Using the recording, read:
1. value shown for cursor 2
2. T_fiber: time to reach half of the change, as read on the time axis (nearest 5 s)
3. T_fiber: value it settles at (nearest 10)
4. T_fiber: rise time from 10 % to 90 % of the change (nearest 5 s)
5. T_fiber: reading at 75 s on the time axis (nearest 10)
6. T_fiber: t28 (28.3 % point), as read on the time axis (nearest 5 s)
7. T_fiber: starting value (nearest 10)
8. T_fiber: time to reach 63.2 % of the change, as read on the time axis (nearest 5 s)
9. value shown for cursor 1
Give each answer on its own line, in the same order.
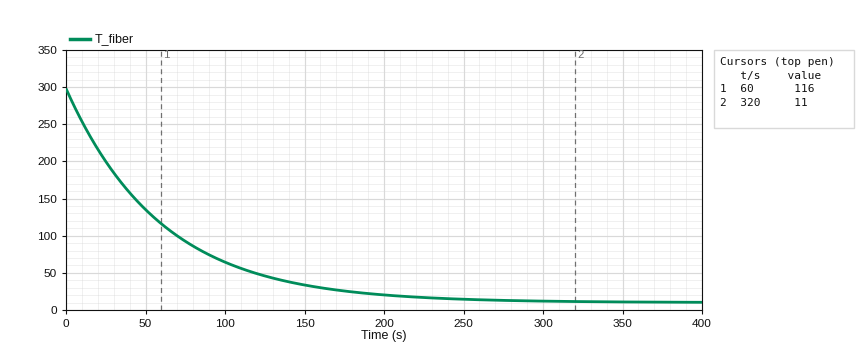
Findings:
11
40 s
10
130 s
90
20 s
300
60 s
116
